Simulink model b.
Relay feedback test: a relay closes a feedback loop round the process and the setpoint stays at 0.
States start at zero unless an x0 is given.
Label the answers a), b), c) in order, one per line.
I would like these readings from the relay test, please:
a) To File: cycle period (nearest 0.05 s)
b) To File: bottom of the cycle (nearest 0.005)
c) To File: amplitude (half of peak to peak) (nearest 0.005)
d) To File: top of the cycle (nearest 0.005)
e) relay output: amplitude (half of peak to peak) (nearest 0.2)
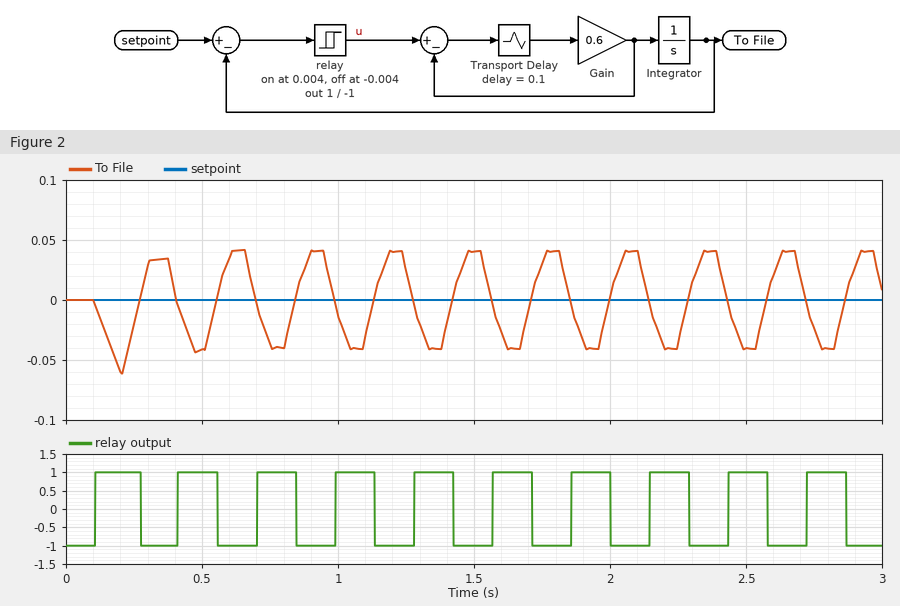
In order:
a) 0.30 s
b) -0.040
c) 0.040
d) 0.040
e) 1.0
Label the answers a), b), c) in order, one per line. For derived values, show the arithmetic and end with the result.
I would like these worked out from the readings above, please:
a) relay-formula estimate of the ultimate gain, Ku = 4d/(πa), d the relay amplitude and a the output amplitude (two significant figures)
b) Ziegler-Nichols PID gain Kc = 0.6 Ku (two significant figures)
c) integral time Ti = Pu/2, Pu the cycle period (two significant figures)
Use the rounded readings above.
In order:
a) 4 × 1 / (π × 0.04) = 32
b) 0.6 × 32 = 19
c) 0.3 / 2 = 0.15 s
